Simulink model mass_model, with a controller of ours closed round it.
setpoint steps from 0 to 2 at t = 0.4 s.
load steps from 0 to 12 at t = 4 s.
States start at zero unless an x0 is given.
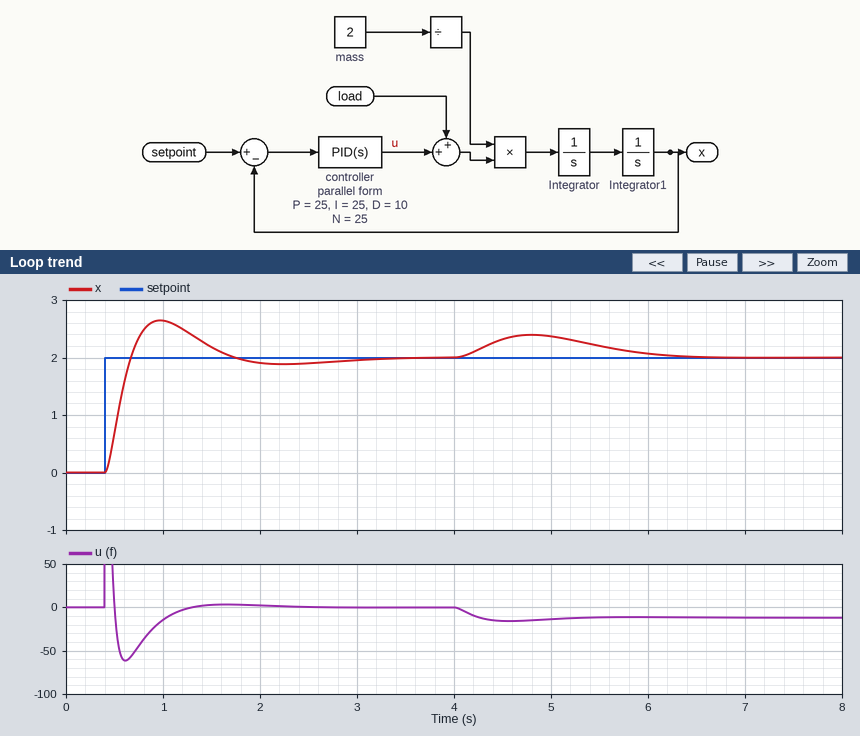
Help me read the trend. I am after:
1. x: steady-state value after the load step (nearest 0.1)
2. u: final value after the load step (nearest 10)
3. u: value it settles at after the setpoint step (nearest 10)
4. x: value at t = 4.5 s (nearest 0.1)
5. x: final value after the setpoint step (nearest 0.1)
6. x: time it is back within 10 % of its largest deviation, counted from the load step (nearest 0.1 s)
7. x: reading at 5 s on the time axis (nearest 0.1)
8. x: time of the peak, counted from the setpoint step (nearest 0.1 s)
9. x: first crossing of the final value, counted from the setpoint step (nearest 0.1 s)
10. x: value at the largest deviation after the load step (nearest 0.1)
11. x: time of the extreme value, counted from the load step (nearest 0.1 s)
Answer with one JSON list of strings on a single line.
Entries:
["2.0", "-10", "0", "2.3", "2.0", "2.2 s", "2.4", "0.6 s", "0.3 s", "2.4", "0.8 s"]
